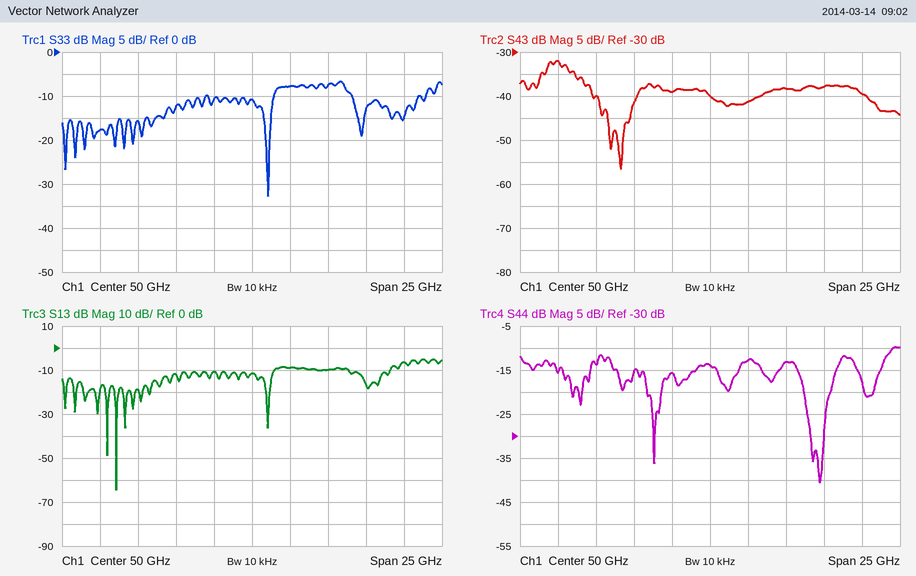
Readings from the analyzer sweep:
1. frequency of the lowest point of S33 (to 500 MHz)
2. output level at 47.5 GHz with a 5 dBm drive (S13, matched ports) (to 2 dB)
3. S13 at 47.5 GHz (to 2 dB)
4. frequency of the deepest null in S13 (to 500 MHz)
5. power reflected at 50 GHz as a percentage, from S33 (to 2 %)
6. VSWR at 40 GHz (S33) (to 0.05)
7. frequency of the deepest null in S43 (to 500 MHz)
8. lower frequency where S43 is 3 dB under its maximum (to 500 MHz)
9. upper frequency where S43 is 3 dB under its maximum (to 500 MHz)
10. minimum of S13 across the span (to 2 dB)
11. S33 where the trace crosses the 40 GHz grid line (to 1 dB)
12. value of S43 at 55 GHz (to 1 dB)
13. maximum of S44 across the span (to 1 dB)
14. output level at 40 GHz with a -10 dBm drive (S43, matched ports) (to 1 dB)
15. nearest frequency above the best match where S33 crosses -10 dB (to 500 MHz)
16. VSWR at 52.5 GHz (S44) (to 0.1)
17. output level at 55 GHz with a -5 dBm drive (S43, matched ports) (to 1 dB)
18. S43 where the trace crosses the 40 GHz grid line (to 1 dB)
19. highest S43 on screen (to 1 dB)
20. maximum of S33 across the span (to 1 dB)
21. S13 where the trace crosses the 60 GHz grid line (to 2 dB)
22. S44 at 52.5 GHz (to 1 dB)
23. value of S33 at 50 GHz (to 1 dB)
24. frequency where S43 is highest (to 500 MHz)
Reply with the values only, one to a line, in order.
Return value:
51.0 GHz
-6 dBm
-10 dB
41.0 GHz
8 %
1.30
44.0 GHz
39.0 GHz
41.0 GHz
-64 dB
-18 dB
-38 dB
-10 dB
-42 dBm
51.5 GHz
1.6
-43 dBm
-32 dB
-32 dB
-7 dB
-6 dB
-13 dB
-11 dB
40.0 GHz
